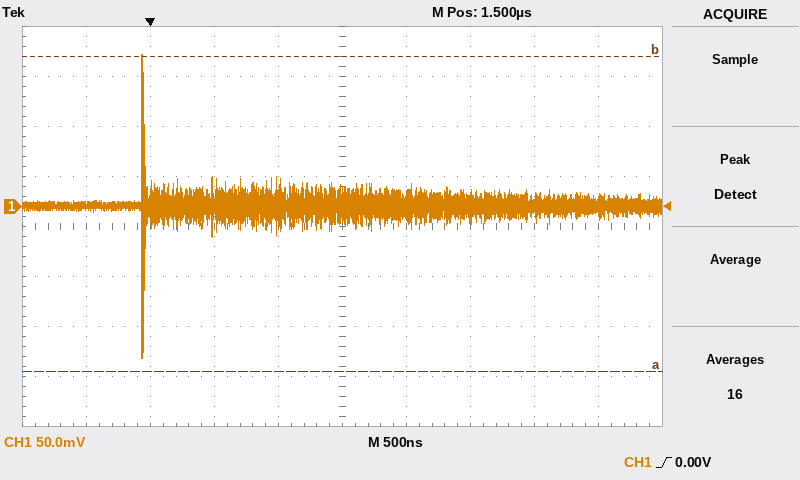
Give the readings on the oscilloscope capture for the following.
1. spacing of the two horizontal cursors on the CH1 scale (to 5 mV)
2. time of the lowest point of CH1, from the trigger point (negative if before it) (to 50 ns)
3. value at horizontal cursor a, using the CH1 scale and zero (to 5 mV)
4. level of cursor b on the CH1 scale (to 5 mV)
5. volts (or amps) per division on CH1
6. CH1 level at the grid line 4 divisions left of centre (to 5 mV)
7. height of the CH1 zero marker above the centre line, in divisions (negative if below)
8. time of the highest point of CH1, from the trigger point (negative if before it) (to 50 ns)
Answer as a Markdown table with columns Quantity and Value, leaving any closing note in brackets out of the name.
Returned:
| Quantity | Value |
|---|---|
| spacing of the two horizontal cursors on the CH1 scale | 315 mV |
| time of the lowest point of CH1, from the trigger point (negative if before it) | -50 ns |
| value at horizontal cursor a, using the CH1 scale and zero | -165 mV |
| level of cursor b on the CH1 scale | 150 mV |
| volts (or amps) per division on CH1 | 50 mV |
| CH1 level at the grid line 4 divisions left of centre | 0 mV |
| height of the CH1 zero marker above the centre line, in divisions | +0.4 div |
| time of the highest point of CH1, from the trigger point (negative if before it) | -50 ns |
